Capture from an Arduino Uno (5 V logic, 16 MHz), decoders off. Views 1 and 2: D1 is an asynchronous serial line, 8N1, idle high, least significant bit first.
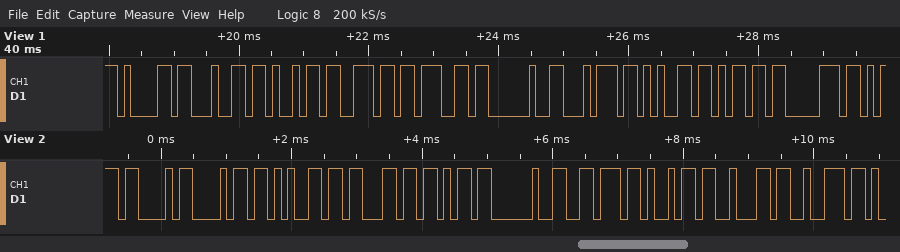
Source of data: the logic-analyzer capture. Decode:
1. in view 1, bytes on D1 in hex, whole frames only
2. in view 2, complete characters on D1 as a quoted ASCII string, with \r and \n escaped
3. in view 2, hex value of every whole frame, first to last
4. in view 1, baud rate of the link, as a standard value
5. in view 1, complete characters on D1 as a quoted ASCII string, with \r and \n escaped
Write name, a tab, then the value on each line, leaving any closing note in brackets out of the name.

in view 1, bytes on D1 in hex, whole frames only	0x61 0x64 0x69 0x6E 0x67 0x20 0x74 0x65 0x6D 0x70
in view 2, complete characters on D1 as a quoted ASCII string, with \r and \n escaped	"Check vibr"
in view 2, hex value of every whole frame, first to last	43 68 65 63 6B 20 76 69 62 72
in view 1, baud rate of the link, as a standard value	9600 baud
in view 1, complete characters on D1 as a quoted ASCII string, with \r and \n escaped	"ading temp"
